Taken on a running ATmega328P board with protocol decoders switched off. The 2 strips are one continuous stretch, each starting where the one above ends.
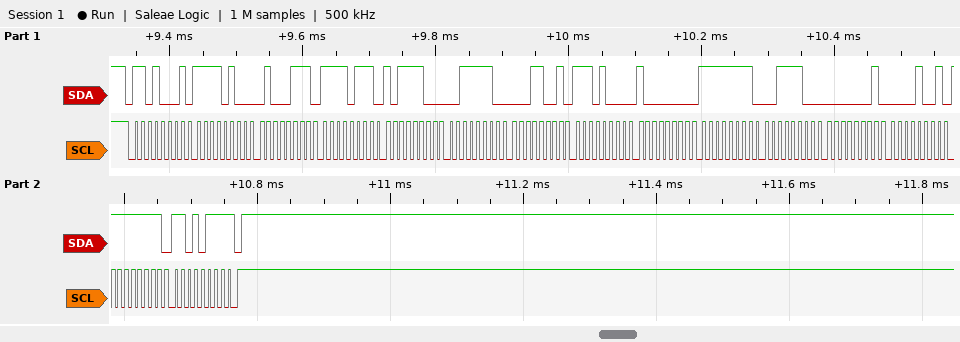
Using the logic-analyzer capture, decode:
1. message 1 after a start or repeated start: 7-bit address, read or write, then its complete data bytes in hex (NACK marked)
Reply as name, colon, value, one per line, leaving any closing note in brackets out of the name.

message 1 after a start or repeated start: 7-bit address, read or write, then its complete data bytes in hex: 0x68 read: F4 47 F7 BC 3E 19 E8 80 FF 3C 01 09 FF D7 NACK
